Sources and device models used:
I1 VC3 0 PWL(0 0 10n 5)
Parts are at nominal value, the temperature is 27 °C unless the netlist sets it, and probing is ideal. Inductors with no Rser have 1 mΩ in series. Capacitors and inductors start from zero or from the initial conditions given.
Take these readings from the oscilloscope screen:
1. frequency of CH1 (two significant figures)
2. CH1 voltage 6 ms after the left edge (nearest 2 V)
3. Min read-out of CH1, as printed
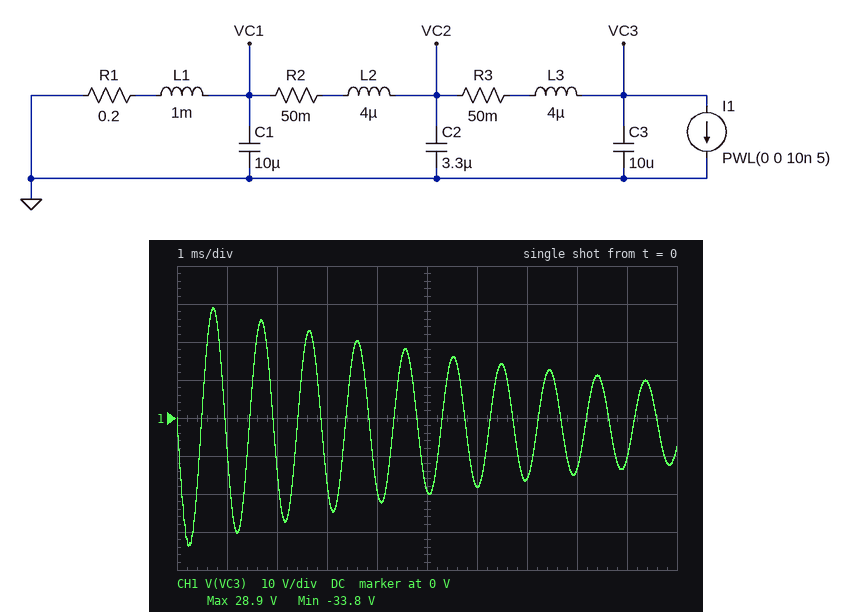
1.0 kHz
-18 V
-33.8 V
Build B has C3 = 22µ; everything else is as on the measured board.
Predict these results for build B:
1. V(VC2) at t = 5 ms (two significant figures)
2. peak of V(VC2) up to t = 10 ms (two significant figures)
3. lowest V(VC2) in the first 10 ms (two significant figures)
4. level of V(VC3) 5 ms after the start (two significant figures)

-15 V
23 V
-27 V
-16 V
